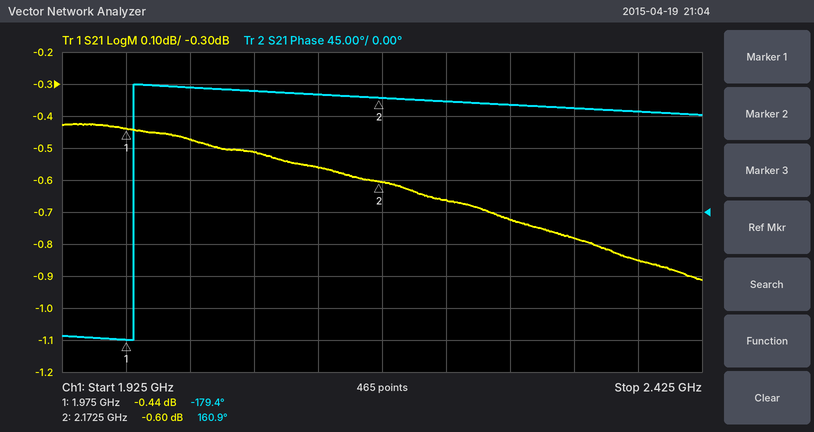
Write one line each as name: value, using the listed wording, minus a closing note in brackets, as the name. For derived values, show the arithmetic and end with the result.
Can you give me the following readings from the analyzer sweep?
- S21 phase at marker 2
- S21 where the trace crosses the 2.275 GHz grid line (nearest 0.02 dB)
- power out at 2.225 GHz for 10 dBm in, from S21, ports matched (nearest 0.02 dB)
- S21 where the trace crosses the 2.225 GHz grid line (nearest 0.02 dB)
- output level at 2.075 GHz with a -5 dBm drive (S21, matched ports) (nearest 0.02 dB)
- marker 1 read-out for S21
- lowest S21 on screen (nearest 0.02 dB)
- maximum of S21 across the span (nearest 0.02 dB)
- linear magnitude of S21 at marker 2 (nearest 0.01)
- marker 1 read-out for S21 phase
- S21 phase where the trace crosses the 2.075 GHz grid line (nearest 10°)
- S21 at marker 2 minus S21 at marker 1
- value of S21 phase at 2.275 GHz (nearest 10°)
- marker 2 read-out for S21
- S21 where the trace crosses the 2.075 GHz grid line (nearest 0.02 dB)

S21 phase at marker 2: 160.9°
S21 where the trace crosses the 2.275 GHz grid line: -0.72 dB
power out at 2.225 GHz for 10 dBm in, from S21, ports matched: 10 dBm + (-0.66 dB) = 9.34 dBm
S21 where the trace crosses the 2.225 GHz grid line: -0.66 dB
output level at 2.075 GHz with a -5 dBm drive (S21, matched ports): -5 dBm + (-0.52 dB) = -5.52 dBm
marker 1 read-out for S21: -0.44 dB
lowest S21 on screen: -0.92 dB
maximum of S21 across the span: -0.42 dB
linear magnitude of S21 at marker 2: 10^(-0.6/20) ≈ 0.93
marker 1 read-out for S21 phase: -179.4°
S21 phase where the trace crosses the 2.075 GHz grid line: 170°
S21 at marker 2 minus S21 at marker 1: -0.6 − (-0.44) = -0.16 dB
value of S21 phase at 2.275 GHz: 150°
marker 2 read-out for S21: -0.60 dB
S21 where the trace crosses the 2.075 GHz grid line: -0.52 dB
